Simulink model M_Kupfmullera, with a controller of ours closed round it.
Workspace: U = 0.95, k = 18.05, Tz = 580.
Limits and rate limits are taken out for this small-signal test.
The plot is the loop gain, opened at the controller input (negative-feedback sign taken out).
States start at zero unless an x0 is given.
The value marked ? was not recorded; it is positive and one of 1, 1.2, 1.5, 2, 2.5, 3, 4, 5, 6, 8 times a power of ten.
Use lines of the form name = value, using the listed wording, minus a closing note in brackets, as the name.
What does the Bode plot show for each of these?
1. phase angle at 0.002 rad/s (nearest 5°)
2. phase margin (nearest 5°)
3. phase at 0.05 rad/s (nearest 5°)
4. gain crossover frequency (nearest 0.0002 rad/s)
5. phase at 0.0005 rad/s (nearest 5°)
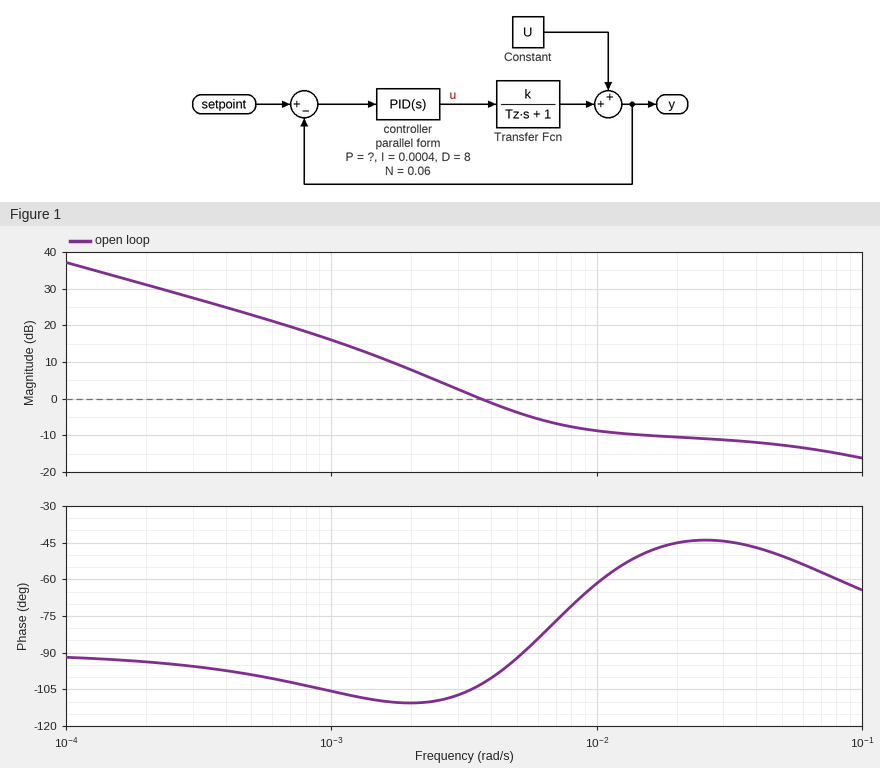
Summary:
phase angle at 0.002 rad/s = -110°
phase margin = 75°
phase at 0.05 rad/s = -50°
gain crossover frequency = 0.0036 rad/s
phase at 0.0005 rad/s = -100°
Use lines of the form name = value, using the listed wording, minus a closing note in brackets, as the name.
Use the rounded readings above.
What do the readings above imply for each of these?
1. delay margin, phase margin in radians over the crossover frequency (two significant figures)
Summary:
delay margin, phase margin in radians over the crossover frequency = 360 s
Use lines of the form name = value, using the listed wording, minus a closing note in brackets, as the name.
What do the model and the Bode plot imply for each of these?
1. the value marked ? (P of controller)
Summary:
the value marked ? = 0.1
